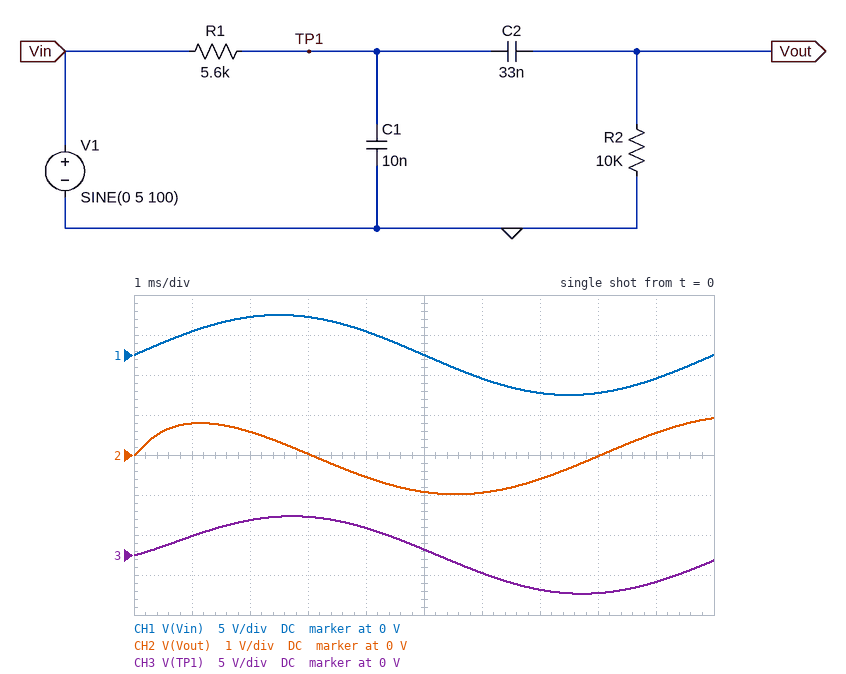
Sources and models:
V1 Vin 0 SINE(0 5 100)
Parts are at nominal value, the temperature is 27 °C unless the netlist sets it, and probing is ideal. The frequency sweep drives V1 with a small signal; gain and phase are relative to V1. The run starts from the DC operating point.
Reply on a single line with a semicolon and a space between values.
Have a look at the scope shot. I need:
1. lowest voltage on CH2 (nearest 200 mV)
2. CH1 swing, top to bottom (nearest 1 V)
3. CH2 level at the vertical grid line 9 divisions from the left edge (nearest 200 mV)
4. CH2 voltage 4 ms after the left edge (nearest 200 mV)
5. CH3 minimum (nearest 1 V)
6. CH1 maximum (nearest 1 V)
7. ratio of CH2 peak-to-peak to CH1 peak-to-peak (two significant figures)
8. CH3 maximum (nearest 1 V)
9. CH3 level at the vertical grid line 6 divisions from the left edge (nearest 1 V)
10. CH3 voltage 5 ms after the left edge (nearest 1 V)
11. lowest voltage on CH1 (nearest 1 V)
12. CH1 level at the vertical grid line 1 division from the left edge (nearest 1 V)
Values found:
-1.0 V; 10 V; 600 mV; -600 mV; -5 V; 5 V; 0.19; 5 V; -2 V; 1 V; -5 V; 3 V
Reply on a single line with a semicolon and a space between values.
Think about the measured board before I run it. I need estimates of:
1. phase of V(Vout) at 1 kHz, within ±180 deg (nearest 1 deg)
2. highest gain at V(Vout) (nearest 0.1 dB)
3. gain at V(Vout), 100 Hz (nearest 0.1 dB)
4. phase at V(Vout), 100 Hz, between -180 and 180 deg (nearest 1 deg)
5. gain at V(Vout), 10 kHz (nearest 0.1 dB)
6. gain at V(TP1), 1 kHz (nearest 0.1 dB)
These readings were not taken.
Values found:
4 deg; -4.8 dB; -14.1 dB; 70 deg; -11.8 dB; -3.9 dB
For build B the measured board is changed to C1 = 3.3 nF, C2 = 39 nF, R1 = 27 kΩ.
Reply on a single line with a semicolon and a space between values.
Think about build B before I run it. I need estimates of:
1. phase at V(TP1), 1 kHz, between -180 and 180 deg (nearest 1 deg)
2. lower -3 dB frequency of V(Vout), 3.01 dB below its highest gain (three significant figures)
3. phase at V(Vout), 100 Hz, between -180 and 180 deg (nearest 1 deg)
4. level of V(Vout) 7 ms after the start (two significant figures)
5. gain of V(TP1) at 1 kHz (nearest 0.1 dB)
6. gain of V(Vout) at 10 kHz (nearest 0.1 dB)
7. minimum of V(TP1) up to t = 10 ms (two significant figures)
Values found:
-24 deg; 102 Hz; 46 deg; -790 mV; -11.2 dB; -16.7 dB; -3.7 V
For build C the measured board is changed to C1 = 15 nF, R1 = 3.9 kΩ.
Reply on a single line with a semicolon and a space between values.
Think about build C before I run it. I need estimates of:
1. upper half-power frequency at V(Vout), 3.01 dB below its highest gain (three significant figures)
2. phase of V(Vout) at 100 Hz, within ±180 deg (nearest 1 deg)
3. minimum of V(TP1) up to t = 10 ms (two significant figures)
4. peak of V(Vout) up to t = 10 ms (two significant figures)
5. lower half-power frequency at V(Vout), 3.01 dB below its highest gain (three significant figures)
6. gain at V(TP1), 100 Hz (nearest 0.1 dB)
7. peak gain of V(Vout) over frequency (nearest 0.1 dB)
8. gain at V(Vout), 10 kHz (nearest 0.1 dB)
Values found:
4.55 kHz; 72 deg; -4.9 V; 940 mV; 288 Hz; -0.2 dB; -3.9 dB; -11.9 dB
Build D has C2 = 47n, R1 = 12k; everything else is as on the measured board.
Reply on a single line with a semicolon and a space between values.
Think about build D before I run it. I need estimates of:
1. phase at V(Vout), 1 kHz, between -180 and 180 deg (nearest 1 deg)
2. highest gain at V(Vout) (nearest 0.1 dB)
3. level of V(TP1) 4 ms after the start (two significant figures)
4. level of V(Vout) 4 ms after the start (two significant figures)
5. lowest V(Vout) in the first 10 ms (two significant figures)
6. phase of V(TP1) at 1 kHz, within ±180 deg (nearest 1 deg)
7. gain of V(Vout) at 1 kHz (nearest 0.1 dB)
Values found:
-10 deg; -7.8 dB; 3.6 V; -390 mV; -1.2 V; -28 deg; -7.9 dB
